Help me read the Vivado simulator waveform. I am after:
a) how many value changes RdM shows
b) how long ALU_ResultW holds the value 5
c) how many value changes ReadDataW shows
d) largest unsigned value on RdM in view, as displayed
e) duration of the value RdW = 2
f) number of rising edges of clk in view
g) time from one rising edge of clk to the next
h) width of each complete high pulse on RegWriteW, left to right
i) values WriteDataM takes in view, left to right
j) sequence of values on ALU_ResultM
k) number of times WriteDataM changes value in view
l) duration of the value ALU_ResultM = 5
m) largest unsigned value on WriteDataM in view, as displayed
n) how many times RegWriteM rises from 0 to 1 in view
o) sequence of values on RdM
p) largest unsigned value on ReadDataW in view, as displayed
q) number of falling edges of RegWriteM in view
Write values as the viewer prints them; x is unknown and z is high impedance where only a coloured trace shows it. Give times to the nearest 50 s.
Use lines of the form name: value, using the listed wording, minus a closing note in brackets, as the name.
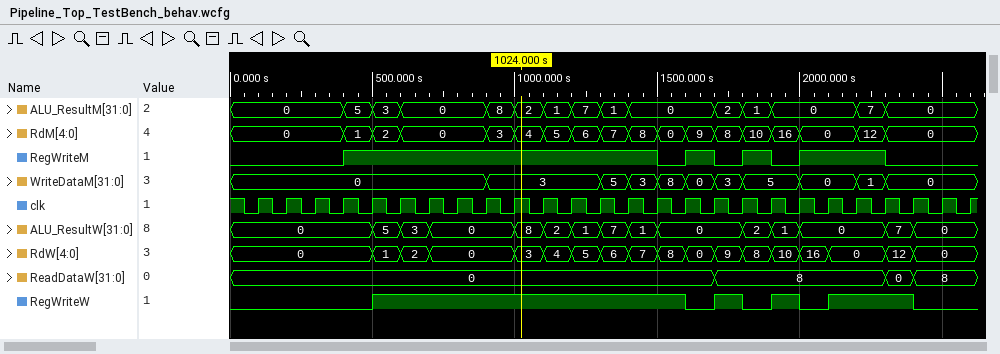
how many value changes RdM shows: 17
how long ALU_ResultW holds the value 5: 100 s
how many value changes ReadDataW shows: 3
largest unsigned value on RdM in view, as displayed: 16
duration of the value RdW = 2: 100 s
number of rising edges of clk in view: 26
time from one rising edge of clk to the next: 100 s
width of each complete high pulse on RegWriteW, left to right: 1100 s, 100 s, 100 s, 300 s
values WriteDataM takes in view, left to right: 0, 3, 5, 3, 8, 0, 3, 5, 0, 1, 0
sequence of values on ALU_ResultM: 0, 5, 3, 0, 8, 2, 1, 7, 1, 0, 2, 1, 0, 7, 0
number of times WriteDataM changes value in view: 10
duration of the value ALU_ResultM = 5: 100 s
largest unsigned value on WriteDataM in view, as displayed: 8
how many times RegWriteM rises from 0 to 1 in view: 4
sequence of values on RdM: 0, 1, 2, 0, 3, 4, 5, 6, 7, 8, 0, 9, 8, 10, 16, 0, 12, 0
largest unsigned value on ReadDataW in view, as displayed: 8
number of falling edges of RegWriteM in view: 4
